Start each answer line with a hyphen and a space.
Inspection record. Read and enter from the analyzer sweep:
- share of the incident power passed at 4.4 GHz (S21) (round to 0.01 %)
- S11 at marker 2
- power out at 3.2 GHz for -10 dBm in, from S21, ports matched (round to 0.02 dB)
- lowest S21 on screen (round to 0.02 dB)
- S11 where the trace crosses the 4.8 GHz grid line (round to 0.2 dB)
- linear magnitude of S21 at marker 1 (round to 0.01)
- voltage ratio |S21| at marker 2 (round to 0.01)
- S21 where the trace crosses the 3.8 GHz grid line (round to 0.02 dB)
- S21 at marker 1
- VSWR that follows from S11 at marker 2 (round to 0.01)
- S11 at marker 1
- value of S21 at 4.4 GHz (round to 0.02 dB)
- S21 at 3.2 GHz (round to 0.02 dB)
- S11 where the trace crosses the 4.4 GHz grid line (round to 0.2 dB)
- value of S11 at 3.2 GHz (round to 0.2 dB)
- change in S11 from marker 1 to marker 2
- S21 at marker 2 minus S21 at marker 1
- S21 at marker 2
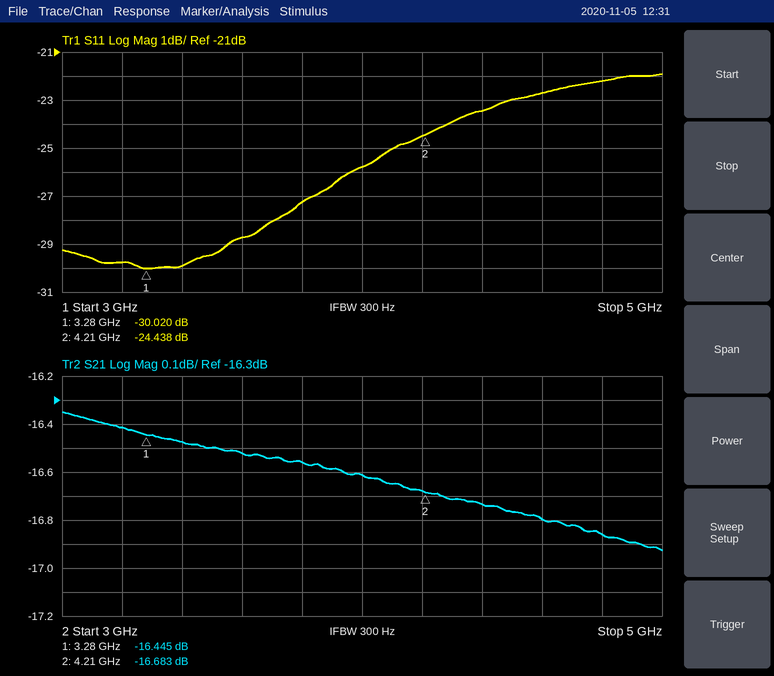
- 2.12 %
- -24.438 dB
- -26.42 dBm
- -16.92 dB
- -22.2 dB
- 0.15
- 0.15
- -16.56 dB
- -16.445 dB
- 1.13
- -30.020 dB
- -16.74 dB
- -16.42 dB
- -23.4 dB
- -29.8 dB
- 5.582 dB
- -0.238 dB
- -16.683 dB
